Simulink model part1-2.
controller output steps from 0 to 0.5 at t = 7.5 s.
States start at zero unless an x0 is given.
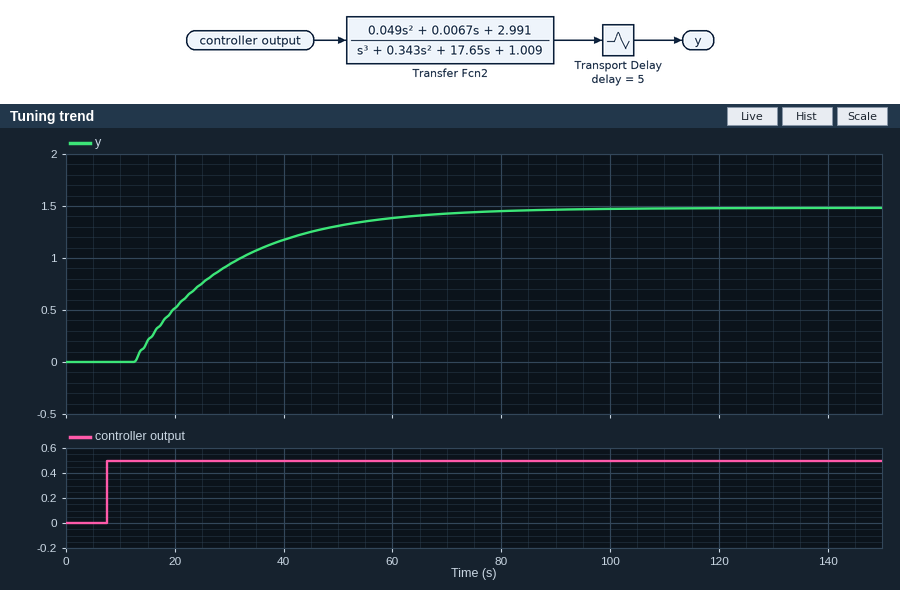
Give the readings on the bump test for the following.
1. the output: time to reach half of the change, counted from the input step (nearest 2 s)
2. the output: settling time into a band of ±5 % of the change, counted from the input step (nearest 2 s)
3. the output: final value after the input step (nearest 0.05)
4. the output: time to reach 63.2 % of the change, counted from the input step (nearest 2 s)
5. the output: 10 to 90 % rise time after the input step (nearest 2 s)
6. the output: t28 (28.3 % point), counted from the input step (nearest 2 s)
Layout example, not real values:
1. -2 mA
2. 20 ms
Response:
1. 18 s
2. 58 s
3. 1.50
4. 22 s
5. 38 s
6. 10 s
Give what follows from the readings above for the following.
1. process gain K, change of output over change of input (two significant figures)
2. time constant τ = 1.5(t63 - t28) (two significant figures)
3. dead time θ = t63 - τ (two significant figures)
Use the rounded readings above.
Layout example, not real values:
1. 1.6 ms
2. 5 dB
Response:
1. 3.0
2. 18 s
3. 4.0 s
